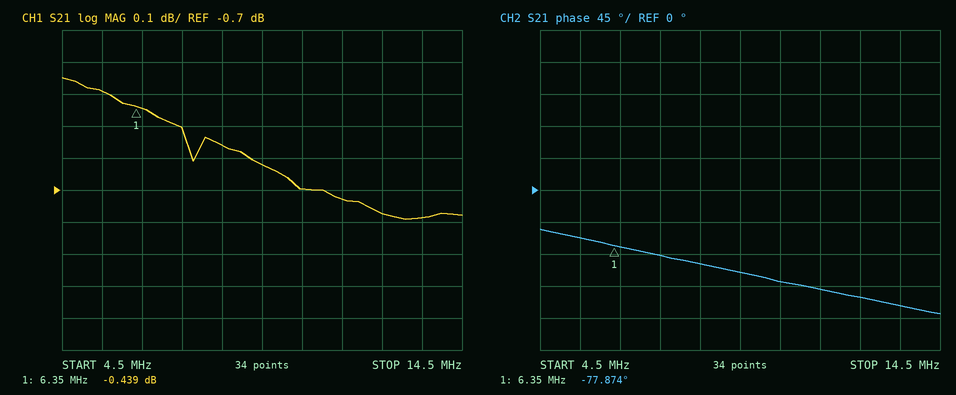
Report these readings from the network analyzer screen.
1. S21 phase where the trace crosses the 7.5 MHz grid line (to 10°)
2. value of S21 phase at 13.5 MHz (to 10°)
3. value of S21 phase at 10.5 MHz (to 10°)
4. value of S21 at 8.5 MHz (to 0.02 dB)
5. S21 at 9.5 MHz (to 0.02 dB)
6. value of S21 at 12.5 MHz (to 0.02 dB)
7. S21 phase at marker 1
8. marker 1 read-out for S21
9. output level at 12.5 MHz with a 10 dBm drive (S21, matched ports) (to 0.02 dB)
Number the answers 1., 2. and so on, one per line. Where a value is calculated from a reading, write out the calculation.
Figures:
1. -90°
2. -160°
3. -130°
4. -0.56 dB
5. -0.62 dB
6. -0.78 dB
7. -77.874°
8. -0.439 dB
9. 10 dBm + (-0.78 dB) = 9.22 dBm
